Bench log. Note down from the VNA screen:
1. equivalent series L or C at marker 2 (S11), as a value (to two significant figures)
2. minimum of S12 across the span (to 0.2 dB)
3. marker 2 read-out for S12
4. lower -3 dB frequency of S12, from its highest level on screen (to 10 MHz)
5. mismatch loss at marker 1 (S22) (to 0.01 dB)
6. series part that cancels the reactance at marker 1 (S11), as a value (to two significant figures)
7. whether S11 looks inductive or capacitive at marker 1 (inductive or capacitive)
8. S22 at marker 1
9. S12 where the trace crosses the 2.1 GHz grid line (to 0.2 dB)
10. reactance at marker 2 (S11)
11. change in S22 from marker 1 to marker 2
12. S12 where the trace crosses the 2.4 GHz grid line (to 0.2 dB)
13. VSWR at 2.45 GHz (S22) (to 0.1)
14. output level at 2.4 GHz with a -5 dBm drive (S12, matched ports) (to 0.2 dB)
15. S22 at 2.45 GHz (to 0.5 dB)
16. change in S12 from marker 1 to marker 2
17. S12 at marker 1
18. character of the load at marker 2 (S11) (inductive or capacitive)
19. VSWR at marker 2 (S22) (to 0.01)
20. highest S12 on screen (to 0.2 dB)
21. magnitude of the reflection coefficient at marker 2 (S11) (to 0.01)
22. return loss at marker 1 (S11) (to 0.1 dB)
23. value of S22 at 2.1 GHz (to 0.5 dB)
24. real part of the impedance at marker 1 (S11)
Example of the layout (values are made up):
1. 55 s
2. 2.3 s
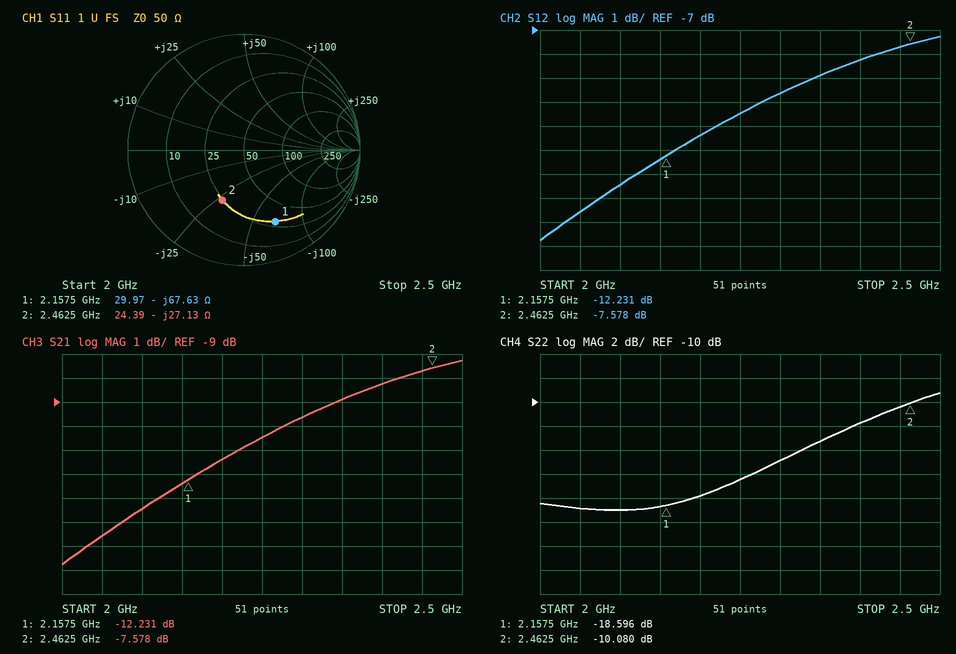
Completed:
1. 2.4 pF
2. -15.8 dB
3. -7.578 dB
4. 2.26 GHz
5. 0.06 dB
6. 5.0 nH
7. capacitive
8. -18.596 dB
9. -13.4 dB
10. -27.13 Ω
11. 8.516 dB
12. -8.2 dB
13. 1.9
14. -13.2 dBm
15. -10.5 dB
16. 4.653 dB
17. -12.231 dB
18. capacitive
19. 1.91
20. -7.2 dB
21. 0.47
22. 3.4 dB
23. -19.0 dB
24. 29.97 Ω
